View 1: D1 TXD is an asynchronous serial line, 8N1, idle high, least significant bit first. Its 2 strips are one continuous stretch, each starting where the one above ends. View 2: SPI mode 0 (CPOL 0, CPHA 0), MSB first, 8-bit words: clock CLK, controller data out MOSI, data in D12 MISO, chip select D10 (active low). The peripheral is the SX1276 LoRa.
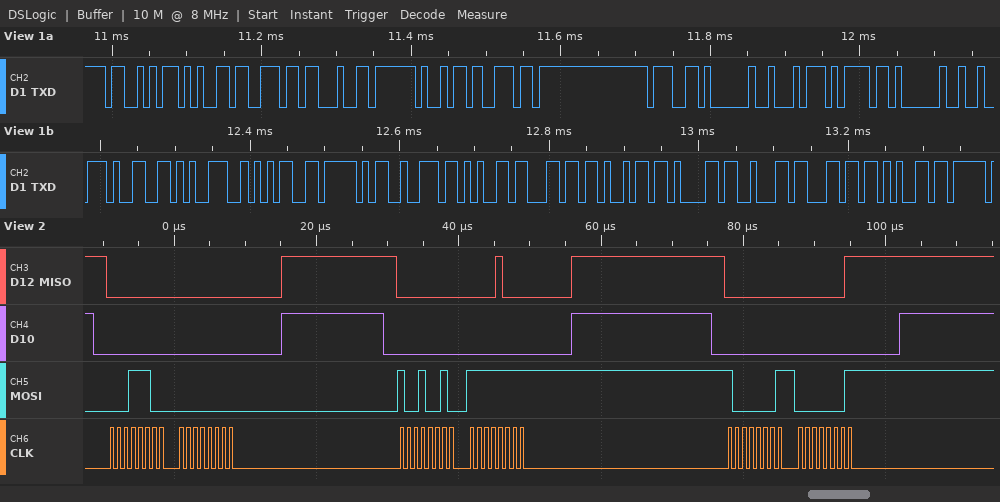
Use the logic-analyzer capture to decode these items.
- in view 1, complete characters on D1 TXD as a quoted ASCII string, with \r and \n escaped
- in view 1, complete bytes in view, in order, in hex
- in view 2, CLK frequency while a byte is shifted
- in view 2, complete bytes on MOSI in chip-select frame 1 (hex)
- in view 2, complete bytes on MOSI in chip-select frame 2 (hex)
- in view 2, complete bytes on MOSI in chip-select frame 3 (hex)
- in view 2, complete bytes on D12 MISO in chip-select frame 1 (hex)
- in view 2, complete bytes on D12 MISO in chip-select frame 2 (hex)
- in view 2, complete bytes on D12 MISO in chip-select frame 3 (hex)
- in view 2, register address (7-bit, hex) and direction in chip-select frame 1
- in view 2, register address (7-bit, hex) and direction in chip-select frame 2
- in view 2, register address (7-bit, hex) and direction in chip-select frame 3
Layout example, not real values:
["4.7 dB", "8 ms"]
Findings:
["\"Sending to rf95_reliable\"", "53 65 6E 64 69 6E 67 20 74 6F 20 72 66 39 35 5F 72 65 6C 69 61 62 6C 65", "1 MHz", "0x1C 0x00", "0x92 0xFF", "0x81 0x01", "0x00 0x00", "0x00 0x08", "0x00 0x01", "0x1C read", "0x12 write", "0x01 write"]
